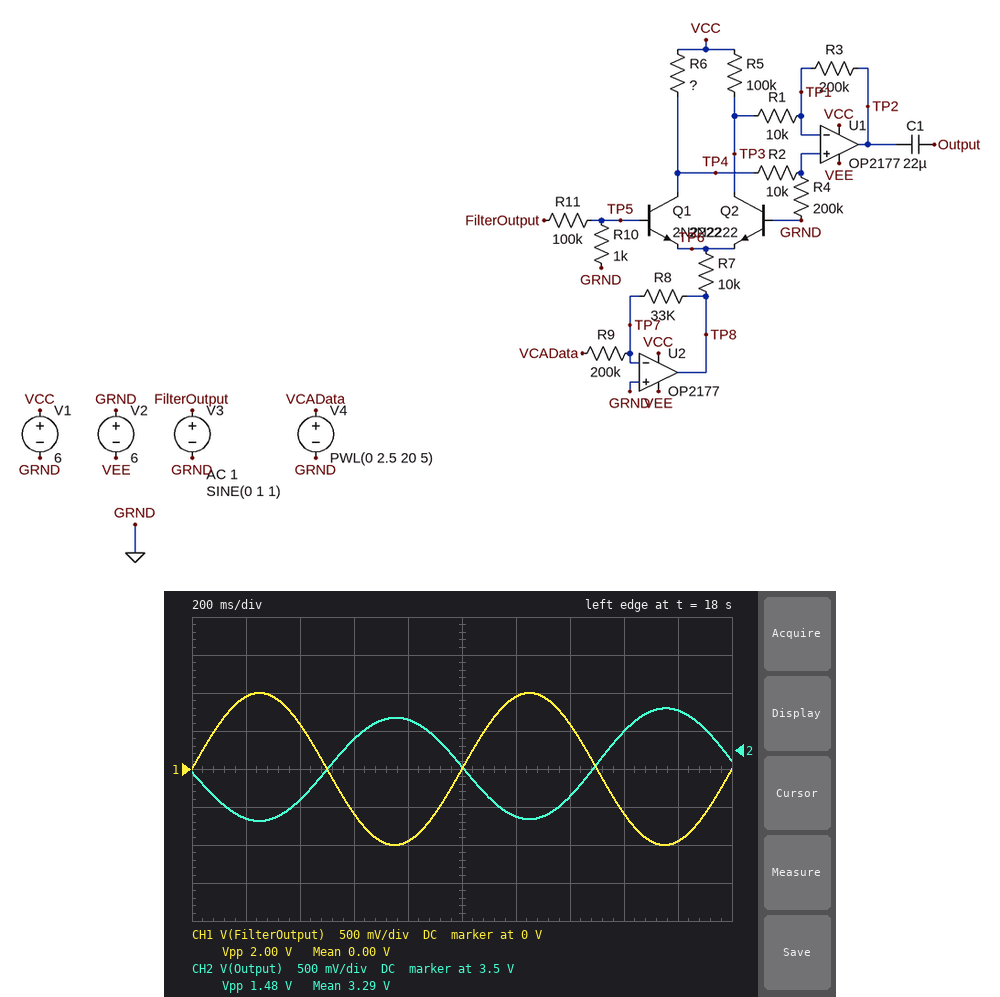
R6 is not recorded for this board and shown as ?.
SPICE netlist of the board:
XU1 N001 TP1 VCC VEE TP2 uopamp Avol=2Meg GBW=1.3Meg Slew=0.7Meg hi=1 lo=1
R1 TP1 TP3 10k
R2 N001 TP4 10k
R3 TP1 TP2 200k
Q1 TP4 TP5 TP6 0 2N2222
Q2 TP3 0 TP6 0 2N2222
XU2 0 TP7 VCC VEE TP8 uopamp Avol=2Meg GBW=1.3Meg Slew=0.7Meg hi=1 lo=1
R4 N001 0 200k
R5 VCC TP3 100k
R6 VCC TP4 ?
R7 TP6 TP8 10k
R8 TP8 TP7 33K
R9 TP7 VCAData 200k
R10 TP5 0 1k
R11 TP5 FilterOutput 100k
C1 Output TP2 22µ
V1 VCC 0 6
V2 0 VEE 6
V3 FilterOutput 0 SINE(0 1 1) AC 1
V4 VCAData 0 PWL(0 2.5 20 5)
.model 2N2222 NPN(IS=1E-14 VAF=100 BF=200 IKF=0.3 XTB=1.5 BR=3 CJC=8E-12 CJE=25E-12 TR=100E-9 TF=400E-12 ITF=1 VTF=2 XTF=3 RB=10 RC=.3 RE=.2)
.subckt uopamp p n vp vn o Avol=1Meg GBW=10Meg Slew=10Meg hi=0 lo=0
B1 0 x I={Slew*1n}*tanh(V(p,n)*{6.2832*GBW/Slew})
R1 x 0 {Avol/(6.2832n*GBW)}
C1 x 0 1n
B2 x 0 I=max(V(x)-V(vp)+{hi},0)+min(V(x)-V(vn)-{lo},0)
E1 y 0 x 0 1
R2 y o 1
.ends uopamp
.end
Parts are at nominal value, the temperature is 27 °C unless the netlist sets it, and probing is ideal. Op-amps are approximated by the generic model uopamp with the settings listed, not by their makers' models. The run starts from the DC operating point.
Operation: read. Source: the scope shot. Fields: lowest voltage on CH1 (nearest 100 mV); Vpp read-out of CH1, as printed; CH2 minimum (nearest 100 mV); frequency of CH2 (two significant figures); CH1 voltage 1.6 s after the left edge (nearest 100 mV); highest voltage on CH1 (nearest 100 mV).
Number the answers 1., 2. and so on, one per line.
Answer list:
1. -1.0 V
2. 2.00 V
3. 2.6 V
4. 1.0 Hz
5. -600 mV
6. 1.0 V
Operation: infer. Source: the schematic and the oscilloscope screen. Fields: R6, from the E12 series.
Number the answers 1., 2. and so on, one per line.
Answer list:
1. 47 kΩ
